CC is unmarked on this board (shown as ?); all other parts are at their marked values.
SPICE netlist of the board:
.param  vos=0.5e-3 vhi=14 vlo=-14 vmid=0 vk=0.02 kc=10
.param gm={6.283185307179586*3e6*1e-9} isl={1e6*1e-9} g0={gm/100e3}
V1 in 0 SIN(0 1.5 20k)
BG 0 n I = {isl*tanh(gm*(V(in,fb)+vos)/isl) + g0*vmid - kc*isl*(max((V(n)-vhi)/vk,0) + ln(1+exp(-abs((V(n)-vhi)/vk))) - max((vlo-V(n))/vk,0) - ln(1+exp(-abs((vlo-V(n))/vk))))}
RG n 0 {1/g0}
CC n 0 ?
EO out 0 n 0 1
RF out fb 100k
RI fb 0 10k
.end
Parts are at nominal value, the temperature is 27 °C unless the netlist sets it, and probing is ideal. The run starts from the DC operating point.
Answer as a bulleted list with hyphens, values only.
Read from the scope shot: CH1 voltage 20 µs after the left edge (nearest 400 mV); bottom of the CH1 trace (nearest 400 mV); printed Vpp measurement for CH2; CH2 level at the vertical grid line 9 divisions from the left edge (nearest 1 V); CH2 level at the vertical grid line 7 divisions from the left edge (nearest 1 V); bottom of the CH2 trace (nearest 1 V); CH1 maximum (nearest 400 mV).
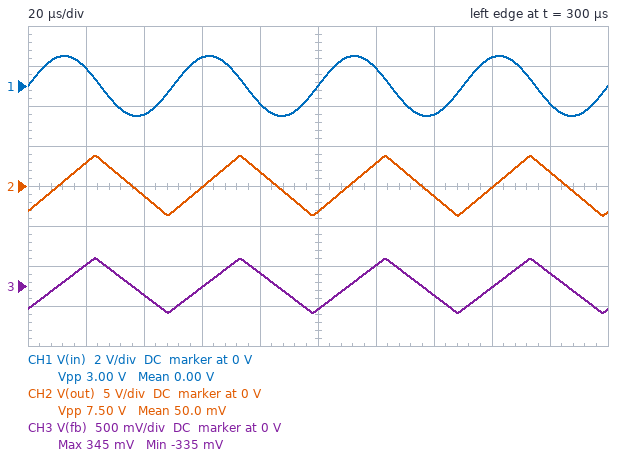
- 800 mV
- -1.6 V
- 7.50 V
- 2 V
- -1 V
- -4 V
- 1.6 V
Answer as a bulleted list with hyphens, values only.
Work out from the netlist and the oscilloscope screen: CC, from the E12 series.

- 3.3 nF
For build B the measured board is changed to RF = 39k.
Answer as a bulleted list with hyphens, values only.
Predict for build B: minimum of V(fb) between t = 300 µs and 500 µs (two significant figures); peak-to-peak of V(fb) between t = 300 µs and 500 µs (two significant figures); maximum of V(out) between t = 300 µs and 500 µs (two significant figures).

- -760 mV
- 1.5 V
- 3.7 V
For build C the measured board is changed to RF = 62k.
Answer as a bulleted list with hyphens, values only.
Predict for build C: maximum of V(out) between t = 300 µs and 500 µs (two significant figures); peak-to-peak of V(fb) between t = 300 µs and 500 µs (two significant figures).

- 3.7 V
- 1.0 V
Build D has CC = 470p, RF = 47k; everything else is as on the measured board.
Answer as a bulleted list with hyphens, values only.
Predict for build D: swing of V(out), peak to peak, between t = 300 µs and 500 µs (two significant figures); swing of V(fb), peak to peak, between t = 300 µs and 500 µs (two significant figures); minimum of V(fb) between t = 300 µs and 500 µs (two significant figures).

- 17 V
- 3.0 V
- -1.5 V
